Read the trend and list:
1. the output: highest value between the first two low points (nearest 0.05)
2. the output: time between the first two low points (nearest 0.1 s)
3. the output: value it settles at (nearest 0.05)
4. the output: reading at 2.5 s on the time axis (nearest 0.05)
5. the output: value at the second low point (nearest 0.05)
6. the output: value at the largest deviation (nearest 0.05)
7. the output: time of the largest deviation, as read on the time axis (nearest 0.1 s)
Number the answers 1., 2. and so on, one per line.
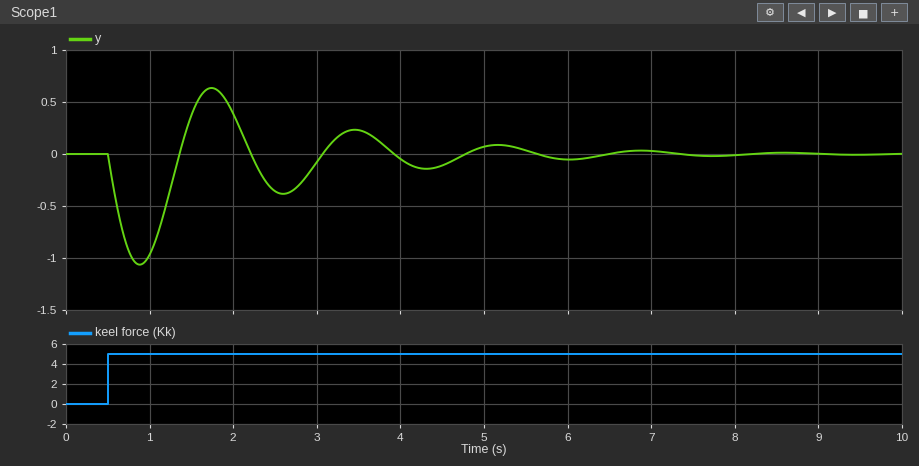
1. 0.65
2. 1.7 s
3. 0.00
4. -0.35
5. -0.40
6. -1.05
7. 0.9 s
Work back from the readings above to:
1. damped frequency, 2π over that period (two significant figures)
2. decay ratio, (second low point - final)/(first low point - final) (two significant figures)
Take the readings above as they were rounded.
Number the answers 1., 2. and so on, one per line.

1. 3.7 rad/s
2. 0.38
